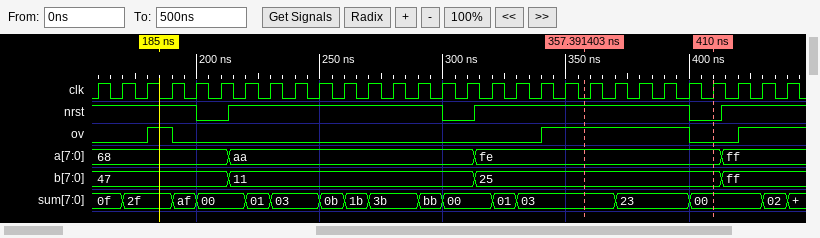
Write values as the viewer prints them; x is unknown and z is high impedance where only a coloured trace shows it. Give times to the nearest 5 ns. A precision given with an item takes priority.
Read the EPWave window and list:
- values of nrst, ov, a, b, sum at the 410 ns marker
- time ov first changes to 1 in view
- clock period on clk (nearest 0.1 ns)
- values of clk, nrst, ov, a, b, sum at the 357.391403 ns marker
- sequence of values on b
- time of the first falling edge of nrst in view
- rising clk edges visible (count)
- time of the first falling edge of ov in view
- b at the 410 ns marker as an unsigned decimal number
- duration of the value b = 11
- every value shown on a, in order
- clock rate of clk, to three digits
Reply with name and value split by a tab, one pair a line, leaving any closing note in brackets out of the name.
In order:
values of nrst, ov, a, b, sum at the 410 ns marker	nrst=0, ov=0, a=fe, b=25, sum=00
time ov first changes to 1 in view	180 ns
clock period on clk	10 ns
values of clk, nrst, ov, a, b, sum at the 357.391403 ns marker	clk=0, nrst=1, ov=1, a=fe, b=25, sum=03
sequence of values on b	47, 11, 25, ff
time of the first falling edge of nrst in view	200 ns
rising clk edges visible	29
time of the first falling edge of ov in view	190 ns
b at the 410 ns marker as an unsigned decimal number	37
duration of the value b = 11	100 ns
every value shown on a, in order	68, aa, fe, ff
clock rate of clk, to three digits	100 MHz
